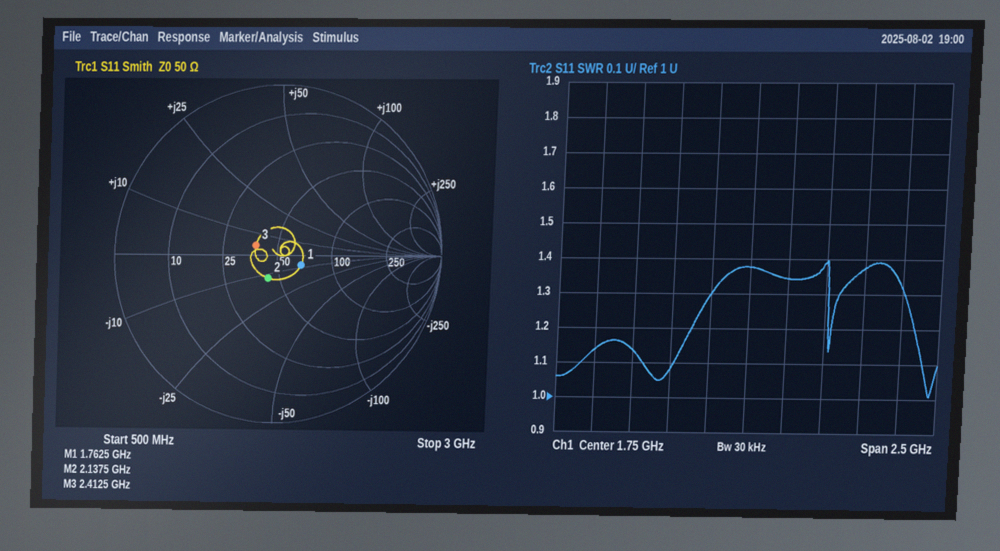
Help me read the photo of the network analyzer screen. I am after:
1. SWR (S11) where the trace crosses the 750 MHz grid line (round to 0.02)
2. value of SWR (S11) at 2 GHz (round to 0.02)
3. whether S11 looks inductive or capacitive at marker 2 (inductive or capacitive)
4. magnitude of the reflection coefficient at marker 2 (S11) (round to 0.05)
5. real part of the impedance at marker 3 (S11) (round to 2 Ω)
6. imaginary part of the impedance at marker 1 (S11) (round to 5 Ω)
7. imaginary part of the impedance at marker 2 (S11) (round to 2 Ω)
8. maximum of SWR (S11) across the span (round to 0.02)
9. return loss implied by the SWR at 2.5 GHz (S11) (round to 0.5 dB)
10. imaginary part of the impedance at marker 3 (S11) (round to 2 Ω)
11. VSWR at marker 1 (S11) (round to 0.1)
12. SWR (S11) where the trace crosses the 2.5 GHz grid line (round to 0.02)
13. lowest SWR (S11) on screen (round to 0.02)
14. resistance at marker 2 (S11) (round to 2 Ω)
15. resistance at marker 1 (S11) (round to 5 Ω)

1.14
1.34
capacitive
0.15
38 Ω
-10 Ω
-12 Ω
1.40
16.0 dB
+4 Ω
1.4
1.38
1.00
44 Ω
65 Ω
